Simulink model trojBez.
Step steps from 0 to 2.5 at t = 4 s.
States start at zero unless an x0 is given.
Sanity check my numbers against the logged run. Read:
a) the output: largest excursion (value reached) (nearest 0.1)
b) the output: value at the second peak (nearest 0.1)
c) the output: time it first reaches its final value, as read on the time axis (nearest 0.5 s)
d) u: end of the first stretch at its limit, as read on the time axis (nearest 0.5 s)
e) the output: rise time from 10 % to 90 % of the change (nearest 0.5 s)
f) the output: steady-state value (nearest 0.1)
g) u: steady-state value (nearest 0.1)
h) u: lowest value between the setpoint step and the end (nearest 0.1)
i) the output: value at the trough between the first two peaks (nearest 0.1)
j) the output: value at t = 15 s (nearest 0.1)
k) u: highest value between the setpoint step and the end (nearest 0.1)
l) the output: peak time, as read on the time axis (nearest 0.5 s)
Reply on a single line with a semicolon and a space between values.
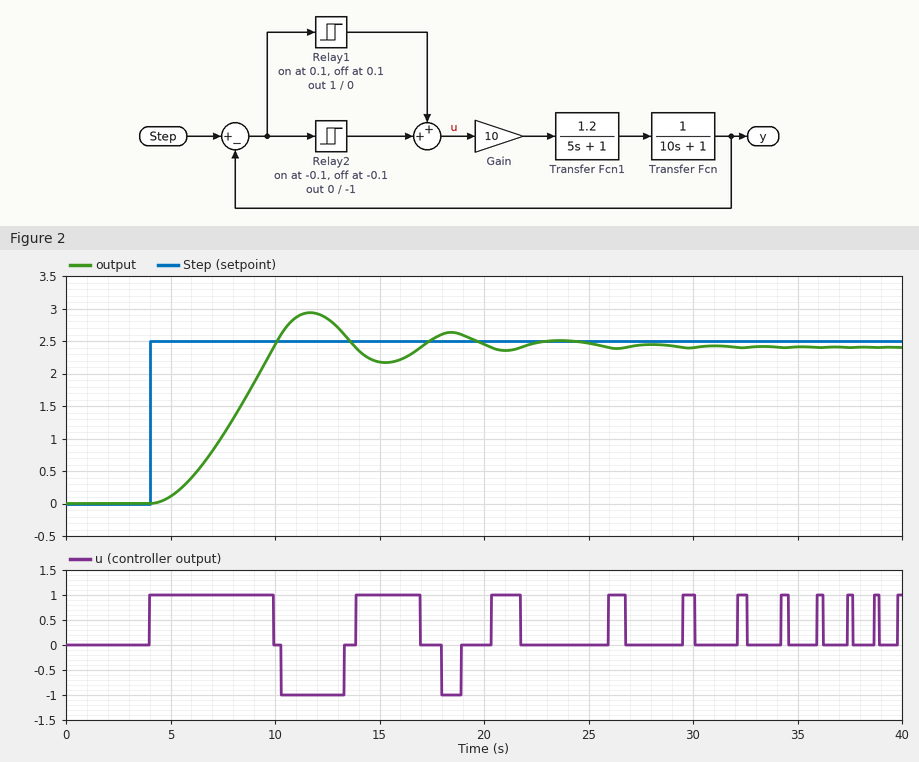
2.9; 2.6; 10.0 s; 10.0 s; 4.0 s; 2.4; 0.0; -1.0; 2.2; 2.2; 1.0; 11.5 s
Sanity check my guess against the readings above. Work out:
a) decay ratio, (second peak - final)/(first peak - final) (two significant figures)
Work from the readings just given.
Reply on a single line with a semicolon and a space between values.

0.40
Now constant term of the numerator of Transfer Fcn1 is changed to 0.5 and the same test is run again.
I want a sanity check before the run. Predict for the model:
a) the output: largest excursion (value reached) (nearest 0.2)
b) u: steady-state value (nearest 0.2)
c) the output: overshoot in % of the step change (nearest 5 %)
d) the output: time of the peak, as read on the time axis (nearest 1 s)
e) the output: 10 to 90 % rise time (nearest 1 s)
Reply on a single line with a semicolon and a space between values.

2.6; 1.0; 10 %; 18 s; 8 s
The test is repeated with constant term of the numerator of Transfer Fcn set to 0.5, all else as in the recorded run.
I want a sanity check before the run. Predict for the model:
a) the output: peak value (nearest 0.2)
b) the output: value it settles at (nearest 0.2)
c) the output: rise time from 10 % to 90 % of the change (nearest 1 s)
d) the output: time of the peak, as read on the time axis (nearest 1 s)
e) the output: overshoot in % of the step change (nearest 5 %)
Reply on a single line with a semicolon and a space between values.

2.6; 2.4; 7 s; 16 s; 10 %
